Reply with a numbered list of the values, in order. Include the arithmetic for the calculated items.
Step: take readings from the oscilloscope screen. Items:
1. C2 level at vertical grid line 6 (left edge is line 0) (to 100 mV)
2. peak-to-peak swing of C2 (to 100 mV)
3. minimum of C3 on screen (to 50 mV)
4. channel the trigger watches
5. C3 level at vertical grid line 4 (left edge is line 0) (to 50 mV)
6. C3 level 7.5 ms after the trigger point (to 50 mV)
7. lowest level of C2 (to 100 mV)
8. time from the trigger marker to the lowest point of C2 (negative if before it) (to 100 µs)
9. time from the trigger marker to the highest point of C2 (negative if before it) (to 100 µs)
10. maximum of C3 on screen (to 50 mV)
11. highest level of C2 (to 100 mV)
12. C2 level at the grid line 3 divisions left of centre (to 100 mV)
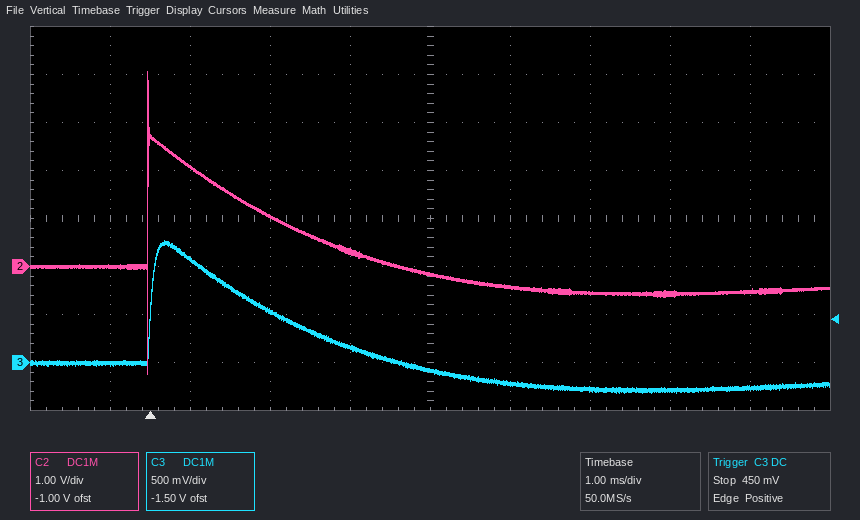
1. -400 mV
2. 4.1 V − (-2.2 V) = 6.3 V
3. -300 mV
4. C3
5. 150 mV
6. -250 mV
7. -2.2 V
8. 0.0 ms
9. 0.0 ms
10. 1.25 V
11. 4.1 V
12. 2.1 V
